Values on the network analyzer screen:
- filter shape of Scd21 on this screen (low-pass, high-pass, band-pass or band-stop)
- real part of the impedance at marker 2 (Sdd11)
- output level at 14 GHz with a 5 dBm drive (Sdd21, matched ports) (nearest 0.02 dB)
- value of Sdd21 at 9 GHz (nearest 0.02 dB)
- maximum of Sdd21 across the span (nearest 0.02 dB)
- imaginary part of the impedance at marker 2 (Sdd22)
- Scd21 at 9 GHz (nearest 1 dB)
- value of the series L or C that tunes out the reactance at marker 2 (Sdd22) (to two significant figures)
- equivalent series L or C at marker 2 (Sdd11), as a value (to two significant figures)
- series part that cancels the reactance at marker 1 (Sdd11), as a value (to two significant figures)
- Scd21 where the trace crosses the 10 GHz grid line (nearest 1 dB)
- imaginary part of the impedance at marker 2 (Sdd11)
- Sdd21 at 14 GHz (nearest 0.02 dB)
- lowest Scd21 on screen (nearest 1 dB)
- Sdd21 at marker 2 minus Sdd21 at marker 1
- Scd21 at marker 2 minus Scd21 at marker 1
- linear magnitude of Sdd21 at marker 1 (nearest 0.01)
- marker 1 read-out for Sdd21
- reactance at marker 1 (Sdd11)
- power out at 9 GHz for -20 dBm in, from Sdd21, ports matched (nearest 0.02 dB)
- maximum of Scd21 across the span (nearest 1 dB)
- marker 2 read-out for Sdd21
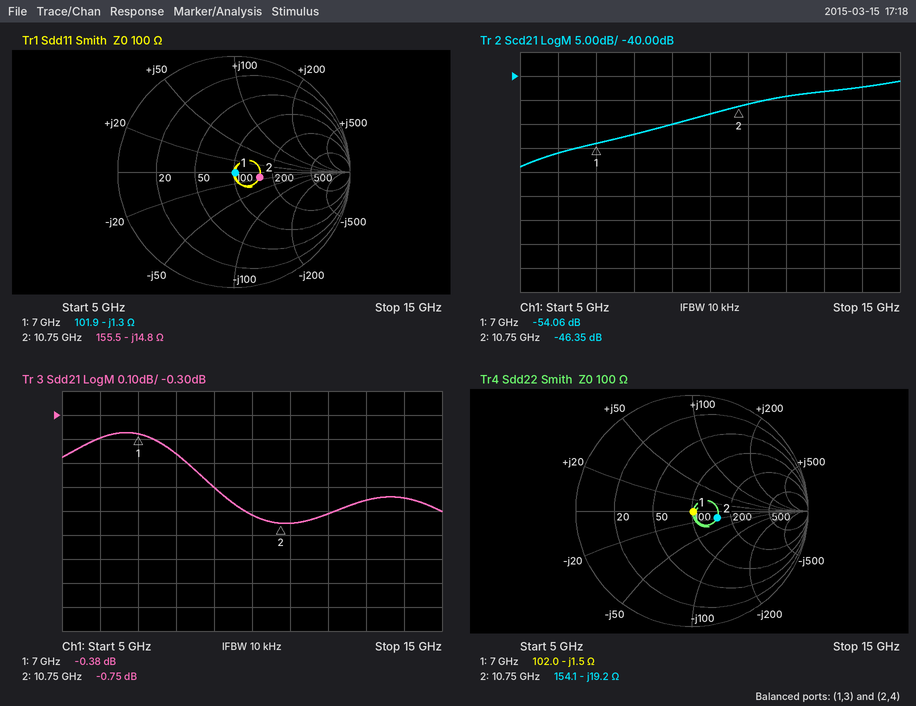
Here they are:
high-pass
155.5 Ω
4.36 dBm
-0.60 dB
-0.38 dB
-19.2 Ω
-50 dB
280 pH
1.00 pF
30 pH
-48 dB
-14.8 Ω
-0.64 dB
-59 dB
-0.37 dB
7.71 dB
0.96
-0.38 dB
-1.3 Ω
-20.60 dBm
-41 dB
-0.75 dB
